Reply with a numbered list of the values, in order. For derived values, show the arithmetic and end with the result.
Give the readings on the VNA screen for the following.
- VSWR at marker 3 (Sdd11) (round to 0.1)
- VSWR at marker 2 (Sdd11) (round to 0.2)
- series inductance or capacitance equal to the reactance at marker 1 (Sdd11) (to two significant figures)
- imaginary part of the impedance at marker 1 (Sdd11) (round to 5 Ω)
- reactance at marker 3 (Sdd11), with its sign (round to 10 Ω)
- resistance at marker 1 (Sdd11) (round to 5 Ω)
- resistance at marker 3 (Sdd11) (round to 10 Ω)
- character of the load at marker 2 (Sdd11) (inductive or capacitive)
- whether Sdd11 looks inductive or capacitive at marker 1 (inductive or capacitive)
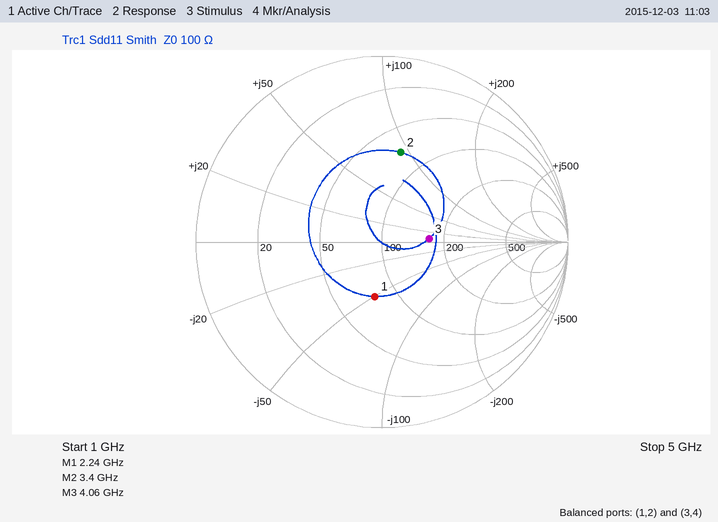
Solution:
1. 1.7
2. 3.0
3. C = 1/(2π × 2.24 GHz × 50 Ω) ≈ 1.4 pF
4. -50 Ω
5. +10 Ω
6. 80 Ω
7. 170 Ω
8. inductive
9. capacitive
